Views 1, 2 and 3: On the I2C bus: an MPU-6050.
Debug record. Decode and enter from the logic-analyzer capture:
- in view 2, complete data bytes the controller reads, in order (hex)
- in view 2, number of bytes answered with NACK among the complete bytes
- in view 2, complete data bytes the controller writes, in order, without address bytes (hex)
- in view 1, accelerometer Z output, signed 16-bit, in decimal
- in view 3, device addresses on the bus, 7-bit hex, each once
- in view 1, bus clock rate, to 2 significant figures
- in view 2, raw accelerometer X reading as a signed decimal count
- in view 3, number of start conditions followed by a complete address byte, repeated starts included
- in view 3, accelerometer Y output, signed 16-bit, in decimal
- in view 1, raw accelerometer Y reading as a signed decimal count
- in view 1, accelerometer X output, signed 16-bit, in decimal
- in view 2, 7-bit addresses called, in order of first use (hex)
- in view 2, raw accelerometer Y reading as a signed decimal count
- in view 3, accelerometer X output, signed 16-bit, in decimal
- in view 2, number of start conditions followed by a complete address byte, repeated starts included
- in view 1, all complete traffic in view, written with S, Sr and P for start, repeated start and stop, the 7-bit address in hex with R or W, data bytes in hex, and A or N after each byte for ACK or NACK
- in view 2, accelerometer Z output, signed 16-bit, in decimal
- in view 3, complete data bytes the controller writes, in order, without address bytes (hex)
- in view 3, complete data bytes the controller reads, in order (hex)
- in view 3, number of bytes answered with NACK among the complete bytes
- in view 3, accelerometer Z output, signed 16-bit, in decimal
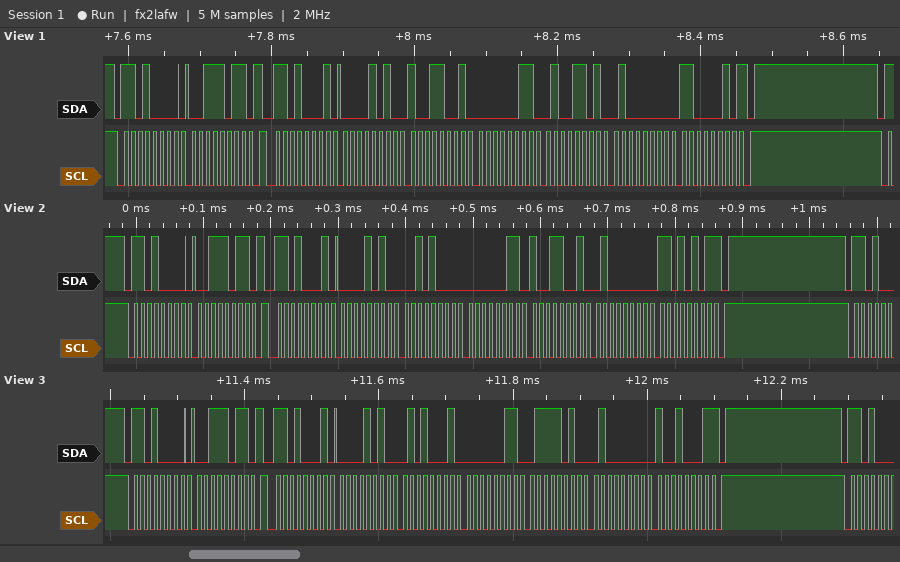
0A 28 03 99 40 D5
1
3B
16578
0x68
100 kHz
2600
2
890
845
2713
0x68
921
2641
2
S 68W A 3B A Sr 68R A 0A A 99 A 03 A 4D A 40 A C2 N P
16597
3B
0A 51 03 7A 40 91
1
16529
